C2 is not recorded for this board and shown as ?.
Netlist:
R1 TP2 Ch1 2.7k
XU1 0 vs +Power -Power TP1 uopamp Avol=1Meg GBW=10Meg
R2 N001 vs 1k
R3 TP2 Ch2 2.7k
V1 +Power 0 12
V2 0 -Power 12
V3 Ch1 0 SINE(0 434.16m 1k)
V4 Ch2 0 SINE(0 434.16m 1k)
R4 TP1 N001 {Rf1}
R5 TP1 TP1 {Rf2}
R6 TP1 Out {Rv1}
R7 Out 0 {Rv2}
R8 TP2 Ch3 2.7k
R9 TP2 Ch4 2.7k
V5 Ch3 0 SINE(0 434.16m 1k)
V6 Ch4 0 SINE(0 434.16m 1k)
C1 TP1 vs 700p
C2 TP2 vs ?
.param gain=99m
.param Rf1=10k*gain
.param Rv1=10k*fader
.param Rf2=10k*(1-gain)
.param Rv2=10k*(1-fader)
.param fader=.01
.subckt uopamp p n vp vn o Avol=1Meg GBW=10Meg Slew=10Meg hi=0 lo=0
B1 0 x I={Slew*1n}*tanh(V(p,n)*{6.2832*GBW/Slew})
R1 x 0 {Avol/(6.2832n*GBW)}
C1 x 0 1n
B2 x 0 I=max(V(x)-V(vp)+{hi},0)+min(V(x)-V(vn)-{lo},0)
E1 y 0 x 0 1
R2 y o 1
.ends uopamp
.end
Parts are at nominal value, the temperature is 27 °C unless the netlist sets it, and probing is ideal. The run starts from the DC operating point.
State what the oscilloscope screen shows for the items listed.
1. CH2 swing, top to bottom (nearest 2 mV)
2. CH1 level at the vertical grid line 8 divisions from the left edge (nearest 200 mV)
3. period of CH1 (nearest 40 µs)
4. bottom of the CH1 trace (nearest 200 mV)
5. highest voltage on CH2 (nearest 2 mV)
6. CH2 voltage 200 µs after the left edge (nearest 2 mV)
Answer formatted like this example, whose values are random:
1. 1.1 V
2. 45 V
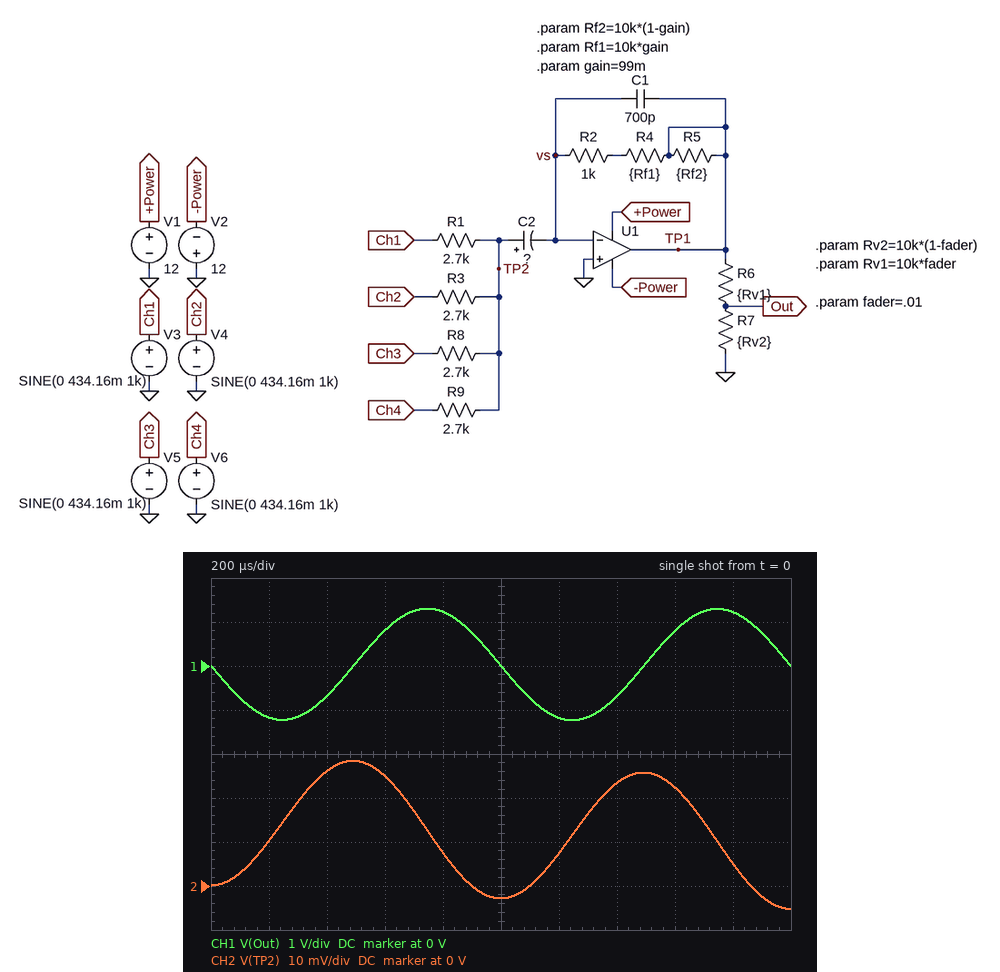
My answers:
1. 34 mV
2. 800 mV
3. 1.00 ms
4. -1.2 V
5. 28 mV
6. 10 mV
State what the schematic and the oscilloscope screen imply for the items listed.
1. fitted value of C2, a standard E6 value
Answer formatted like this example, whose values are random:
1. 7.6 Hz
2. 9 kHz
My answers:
1. 6.8 µF
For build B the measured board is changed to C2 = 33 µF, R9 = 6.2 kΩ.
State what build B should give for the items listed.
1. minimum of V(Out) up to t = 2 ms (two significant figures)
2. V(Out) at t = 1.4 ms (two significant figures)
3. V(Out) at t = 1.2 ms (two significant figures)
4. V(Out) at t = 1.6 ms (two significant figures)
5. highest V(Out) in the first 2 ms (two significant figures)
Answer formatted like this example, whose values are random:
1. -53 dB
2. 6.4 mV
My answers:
1. -1.1 V
2. -640 mV
3. -1.0 V
4. 640 mV
5. 1.1 V
